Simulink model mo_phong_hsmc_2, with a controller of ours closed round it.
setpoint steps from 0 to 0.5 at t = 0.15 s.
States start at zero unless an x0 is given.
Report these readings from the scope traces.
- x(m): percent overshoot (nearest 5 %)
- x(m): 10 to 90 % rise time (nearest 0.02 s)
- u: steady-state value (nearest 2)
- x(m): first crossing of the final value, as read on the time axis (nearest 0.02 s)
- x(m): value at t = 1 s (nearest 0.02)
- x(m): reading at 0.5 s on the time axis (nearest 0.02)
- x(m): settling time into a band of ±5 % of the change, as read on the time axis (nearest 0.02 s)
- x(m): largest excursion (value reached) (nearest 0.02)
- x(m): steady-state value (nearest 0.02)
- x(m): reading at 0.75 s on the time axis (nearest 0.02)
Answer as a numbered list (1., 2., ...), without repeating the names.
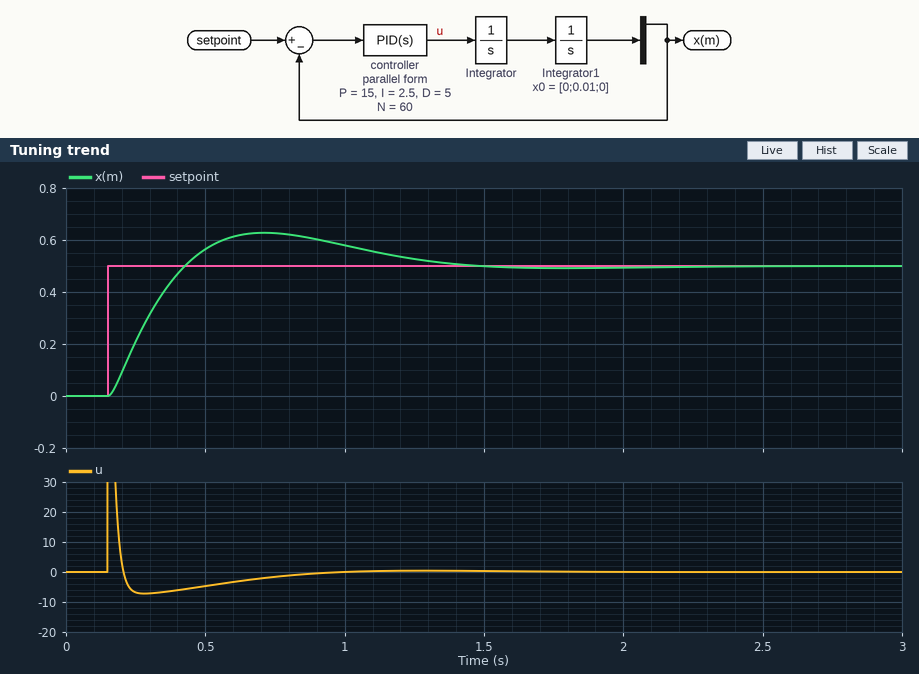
1. 25 %
2. 0.20 s
3. 0
4. 0.42 s
5. 0.58
6. 0.56
7. 1.26 s
8. 0.62
9. 0.50
10. 0.62
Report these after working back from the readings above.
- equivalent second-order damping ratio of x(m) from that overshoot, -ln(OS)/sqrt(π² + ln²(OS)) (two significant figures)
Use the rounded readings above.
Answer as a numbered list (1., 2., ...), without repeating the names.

1. 0.40
